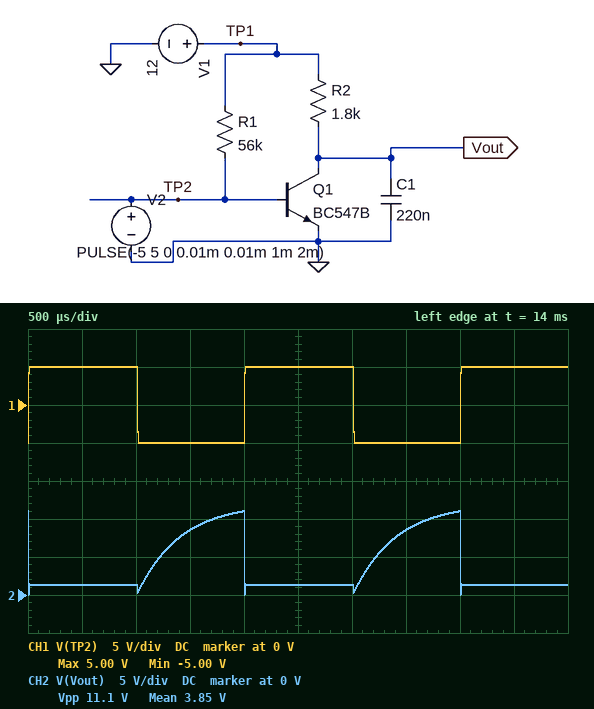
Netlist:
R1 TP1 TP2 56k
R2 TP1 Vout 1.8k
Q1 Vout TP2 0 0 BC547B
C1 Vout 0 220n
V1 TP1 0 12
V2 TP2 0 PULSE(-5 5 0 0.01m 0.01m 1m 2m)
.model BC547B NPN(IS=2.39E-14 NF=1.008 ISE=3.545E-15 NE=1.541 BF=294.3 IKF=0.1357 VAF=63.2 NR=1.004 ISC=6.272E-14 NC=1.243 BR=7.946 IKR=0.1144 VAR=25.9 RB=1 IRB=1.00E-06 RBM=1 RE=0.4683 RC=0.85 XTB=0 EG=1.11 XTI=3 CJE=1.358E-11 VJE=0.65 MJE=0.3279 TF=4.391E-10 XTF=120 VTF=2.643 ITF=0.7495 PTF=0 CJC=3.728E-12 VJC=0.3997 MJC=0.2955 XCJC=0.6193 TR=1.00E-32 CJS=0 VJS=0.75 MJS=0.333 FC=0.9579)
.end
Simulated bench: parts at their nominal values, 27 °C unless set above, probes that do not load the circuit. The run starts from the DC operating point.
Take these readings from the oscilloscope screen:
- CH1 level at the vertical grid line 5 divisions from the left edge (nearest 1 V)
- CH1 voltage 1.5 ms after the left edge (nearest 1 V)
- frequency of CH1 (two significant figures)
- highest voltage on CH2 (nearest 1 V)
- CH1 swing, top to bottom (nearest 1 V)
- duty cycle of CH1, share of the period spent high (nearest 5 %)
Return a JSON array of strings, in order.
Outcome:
["5 V", "-5 V", "500 Hz", "11 V", "10 V", "50 %"]
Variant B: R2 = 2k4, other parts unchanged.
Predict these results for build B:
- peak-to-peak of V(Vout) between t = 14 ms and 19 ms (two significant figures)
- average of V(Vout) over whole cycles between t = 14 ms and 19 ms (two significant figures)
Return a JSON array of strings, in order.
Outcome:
["10 V", "4.0 V"]
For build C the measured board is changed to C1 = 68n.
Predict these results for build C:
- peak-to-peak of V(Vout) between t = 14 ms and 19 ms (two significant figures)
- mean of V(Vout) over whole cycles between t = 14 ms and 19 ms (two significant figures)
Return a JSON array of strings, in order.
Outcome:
["12 V", "5.9 V"]
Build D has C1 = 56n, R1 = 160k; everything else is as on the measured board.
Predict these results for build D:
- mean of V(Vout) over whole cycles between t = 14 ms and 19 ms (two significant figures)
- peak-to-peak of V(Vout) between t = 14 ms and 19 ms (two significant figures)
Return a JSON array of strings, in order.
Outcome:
["6.0 V", "12 V"]
